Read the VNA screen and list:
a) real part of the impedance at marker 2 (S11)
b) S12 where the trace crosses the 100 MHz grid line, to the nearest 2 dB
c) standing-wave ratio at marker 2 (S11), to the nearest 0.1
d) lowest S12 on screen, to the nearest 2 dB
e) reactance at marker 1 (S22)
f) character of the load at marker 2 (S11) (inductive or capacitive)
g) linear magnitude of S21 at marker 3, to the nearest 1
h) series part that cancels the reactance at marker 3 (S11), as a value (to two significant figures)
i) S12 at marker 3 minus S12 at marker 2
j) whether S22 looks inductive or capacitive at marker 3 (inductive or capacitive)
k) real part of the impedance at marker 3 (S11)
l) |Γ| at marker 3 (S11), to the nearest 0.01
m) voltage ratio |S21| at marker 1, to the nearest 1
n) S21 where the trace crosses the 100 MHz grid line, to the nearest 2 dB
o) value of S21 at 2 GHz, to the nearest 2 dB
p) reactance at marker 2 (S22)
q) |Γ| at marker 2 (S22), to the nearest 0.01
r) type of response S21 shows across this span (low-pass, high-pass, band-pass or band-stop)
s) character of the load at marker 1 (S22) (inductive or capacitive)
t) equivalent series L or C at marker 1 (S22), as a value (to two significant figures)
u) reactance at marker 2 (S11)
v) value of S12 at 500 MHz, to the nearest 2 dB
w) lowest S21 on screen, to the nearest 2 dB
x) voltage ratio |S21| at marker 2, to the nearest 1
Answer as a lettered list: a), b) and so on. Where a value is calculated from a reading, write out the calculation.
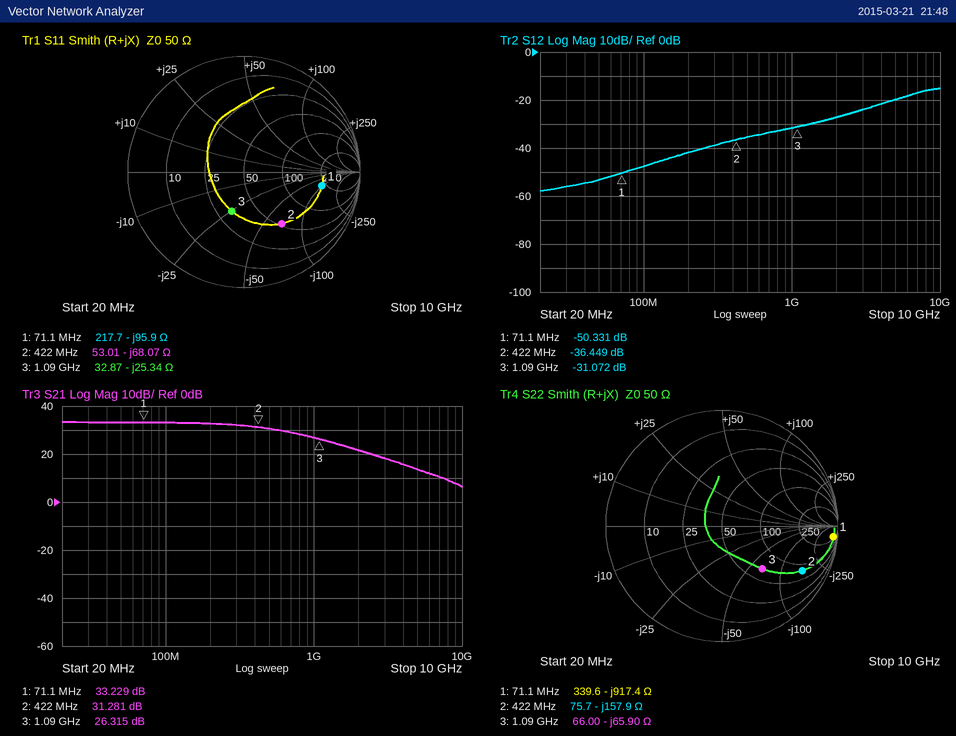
a) 53.01 Ω
b) -48 dB
c) 3.5
d) -58 dB
e) -917.4 Ω
f) capacitive
g) 10^(26.315/20) ≈ 21
h) L = 25.34 Ω/(2π × 1.09 GHz) ≈ 3.7 nH
i) -31.072 − (-36.449) = 5.377 dB
j) capacitive
k) 32.87 Ω
l) 0.35
m) 10^(33.229/20) ≈ 46
n) 34 dB
o) 22 dB
p) -157.9 Ω
q) 0.79
r) low-pass
s) capacitive
t) C = 1/(2π × 71.1 MHz × 917.4 Ω) ≈ 2.4 pF
u) -68.07 Ω
v) -36 dB
w) 6 dB
x) 10^(31.281/20) ≈ 37
